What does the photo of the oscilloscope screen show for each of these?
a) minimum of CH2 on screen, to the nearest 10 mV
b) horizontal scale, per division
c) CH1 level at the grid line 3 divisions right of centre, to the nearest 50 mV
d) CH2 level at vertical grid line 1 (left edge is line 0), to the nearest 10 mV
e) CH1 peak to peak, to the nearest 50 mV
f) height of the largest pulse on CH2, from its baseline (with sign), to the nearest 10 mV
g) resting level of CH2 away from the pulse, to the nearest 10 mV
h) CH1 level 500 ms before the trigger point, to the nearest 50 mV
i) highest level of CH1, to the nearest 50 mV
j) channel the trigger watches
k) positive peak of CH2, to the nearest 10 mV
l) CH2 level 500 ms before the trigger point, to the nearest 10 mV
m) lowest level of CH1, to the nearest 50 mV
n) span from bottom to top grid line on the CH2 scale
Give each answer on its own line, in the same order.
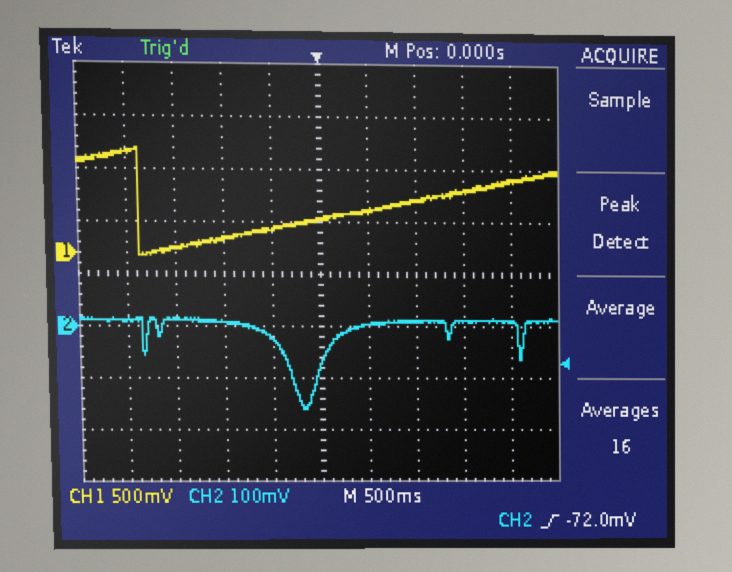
-160 mV
500 ms
600 mV
10 mV
1.00 V
-170 mV
10 mV
250 mV
1.00 V
CH2
20 mV
-20 mV
0 mV
800 mV
